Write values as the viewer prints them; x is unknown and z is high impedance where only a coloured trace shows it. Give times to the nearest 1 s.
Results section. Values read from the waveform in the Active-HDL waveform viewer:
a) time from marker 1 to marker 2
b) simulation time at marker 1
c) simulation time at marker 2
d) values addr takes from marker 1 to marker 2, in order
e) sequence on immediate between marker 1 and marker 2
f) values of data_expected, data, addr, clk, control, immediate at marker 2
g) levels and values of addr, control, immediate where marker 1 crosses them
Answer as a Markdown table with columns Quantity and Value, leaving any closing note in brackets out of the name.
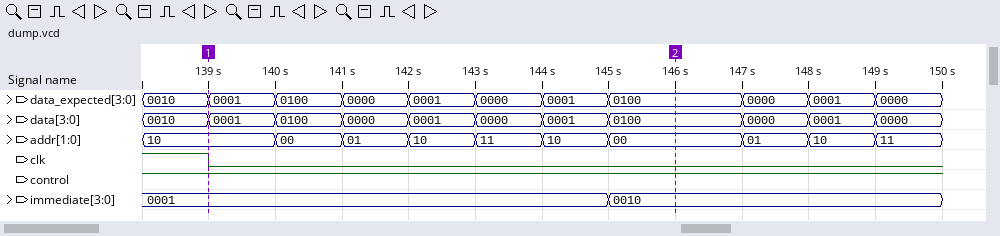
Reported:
| Quantity | Value |
|---|---|
| time from marker 1 to marker 2 | 7 s |
| simulation time at marker 1 | 139 s |
| simulation time at marker 2 | 146 s |
| values addr takes from marker 1 to marker 2, in order | 10, 00, 01, 10, 11, 10, 00 |
| sequence on immediate between marker 1 and marker 2 | 0001, 0010 |
| values of data_expected, data, addr, clk, control, immediate at marker 2 | data_expected=0100, data=0100, addr=00, clk=0, control=1, immediate=0010 |
| levels and values of addr, control, immediate where marker 1 crosses them | addr=10, control=1, immediate=0001 |
